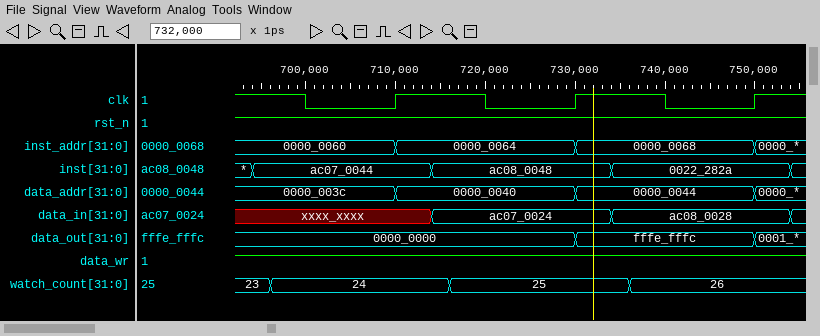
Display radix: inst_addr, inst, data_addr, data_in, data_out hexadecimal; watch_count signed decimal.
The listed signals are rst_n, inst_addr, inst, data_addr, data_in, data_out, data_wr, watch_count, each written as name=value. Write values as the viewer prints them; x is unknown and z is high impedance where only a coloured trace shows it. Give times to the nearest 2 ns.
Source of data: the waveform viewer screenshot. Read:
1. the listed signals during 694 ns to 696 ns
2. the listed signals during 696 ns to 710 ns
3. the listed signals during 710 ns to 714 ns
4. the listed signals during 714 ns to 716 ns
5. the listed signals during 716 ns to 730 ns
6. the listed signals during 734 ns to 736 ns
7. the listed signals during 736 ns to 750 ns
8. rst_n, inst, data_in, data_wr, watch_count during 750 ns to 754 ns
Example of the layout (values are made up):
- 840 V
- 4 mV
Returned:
- rst_n=1, inst_addr=0000_0060, inst=ac07_0044, data_addr=0000_003c, data_in=xxxx_xxxx, data_out=0000_0000, data_wr=1, watch_count=23
- rst_n=1, inst_addr=0000_0060, inst=ac07_0044, data_addr=0000_003c, data_in=xxxx_xxxx, data_out=0000_0000, data_wr=1, watch_count=24
- rst_n=1, inst_addr=0000_0064, inst=ac07_0044, data_addr=0000_0040, data_in=xxxx_xxxx, data_out=0000_0000, data_wr=1, watch_count=24
- rst_n=1, inst_addr=0000_0064, inst=ac08_0048, data_addr=0000_0040, data_in=ac07_0024, data_out=0000_0000, data_wr=1, watch_count=24
- rst_n=1, inst_addr=0000_0064, inst=ac08_0048, data_addr=0000_0040, data_in=ac07_0024, data_out=0000_0000, data_wr=1, watch_count=25
- rst_n=1, inst_addr=0000_0068, inst=0022_282a, data_addr=0000_0044, data_in=ac08_0028, data_out=fffe_fffc, data_wr=1, watch_count=25
- rst_n=1, inst_addr=0000_0068, inst=0022_282a, data_addr=0000_0044, data_in=ac08_0028, data_out=fffe_fffc, data_wr=1, watch_count=26
- rst_n=1, inst=0022_282a, data_in=ac08_0028, data_wr=1, watch_count=26
